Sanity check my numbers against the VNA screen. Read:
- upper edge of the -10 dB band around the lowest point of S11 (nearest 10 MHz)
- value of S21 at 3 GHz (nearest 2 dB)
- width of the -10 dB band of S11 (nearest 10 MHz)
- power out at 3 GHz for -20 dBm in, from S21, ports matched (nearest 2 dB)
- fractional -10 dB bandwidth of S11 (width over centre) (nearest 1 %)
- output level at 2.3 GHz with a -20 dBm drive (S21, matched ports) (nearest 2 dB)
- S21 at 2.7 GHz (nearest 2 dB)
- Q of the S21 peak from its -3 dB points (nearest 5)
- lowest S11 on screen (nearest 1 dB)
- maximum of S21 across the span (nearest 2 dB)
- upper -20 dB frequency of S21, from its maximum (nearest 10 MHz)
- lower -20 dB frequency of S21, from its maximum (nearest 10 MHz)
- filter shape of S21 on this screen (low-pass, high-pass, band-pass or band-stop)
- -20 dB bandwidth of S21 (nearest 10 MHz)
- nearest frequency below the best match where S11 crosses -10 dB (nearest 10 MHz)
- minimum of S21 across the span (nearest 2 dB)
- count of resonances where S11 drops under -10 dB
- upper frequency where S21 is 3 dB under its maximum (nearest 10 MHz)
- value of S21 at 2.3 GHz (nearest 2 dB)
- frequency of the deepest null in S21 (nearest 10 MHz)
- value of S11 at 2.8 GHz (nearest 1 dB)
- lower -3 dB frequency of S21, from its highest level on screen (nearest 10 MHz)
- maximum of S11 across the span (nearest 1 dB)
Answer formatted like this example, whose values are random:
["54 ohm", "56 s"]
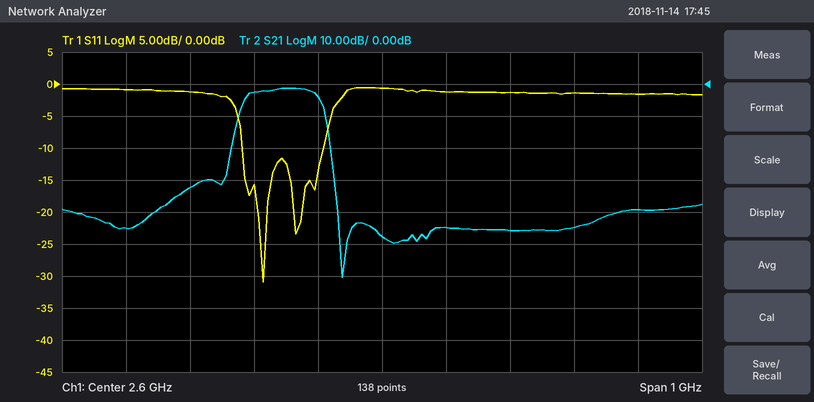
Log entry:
["2.51 GHz", "-40 dB", "130 MHz", "-60 dBm", "5 %", "-52 dBm", "-44 dB", "20", "-31 dB", "-2 dB", "2.52 GHz", "2.36 GHz", "band-pass", "160 MHz", "2.38 GHz", "-60 dB", "2", "2.50 GHz", "-32 dB", "2.54 GHz", "-1 dB", "2.39 GHz", "-1 dB"]
